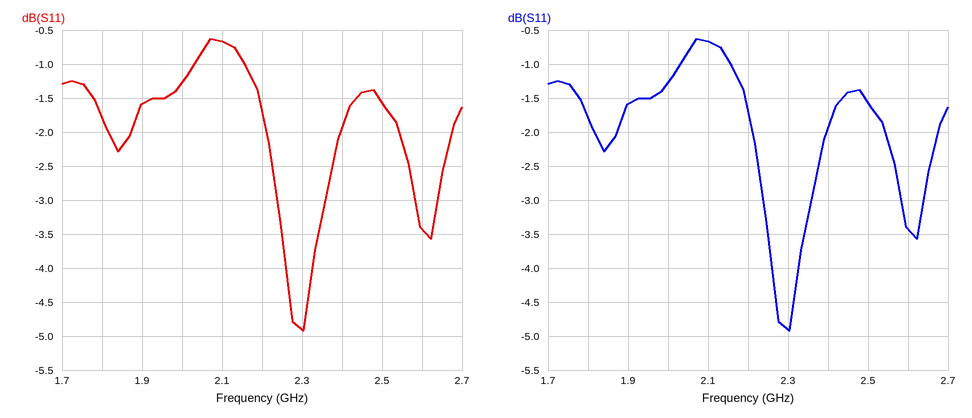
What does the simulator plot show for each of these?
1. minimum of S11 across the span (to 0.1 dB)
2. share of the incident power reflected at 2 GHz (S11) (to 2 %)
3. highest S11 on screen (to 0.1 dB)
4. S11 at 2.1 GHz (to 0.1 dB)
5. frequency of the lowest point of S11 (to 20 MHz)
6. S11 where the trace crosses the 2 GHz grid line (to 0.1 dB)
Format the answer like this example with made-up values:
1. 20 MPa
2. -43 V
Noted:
1. -4.9 dB
2. 74 %
3. -0.6 dB
4. -0.7 dB
5. 2.30 GHz
6. -1.3 dB
